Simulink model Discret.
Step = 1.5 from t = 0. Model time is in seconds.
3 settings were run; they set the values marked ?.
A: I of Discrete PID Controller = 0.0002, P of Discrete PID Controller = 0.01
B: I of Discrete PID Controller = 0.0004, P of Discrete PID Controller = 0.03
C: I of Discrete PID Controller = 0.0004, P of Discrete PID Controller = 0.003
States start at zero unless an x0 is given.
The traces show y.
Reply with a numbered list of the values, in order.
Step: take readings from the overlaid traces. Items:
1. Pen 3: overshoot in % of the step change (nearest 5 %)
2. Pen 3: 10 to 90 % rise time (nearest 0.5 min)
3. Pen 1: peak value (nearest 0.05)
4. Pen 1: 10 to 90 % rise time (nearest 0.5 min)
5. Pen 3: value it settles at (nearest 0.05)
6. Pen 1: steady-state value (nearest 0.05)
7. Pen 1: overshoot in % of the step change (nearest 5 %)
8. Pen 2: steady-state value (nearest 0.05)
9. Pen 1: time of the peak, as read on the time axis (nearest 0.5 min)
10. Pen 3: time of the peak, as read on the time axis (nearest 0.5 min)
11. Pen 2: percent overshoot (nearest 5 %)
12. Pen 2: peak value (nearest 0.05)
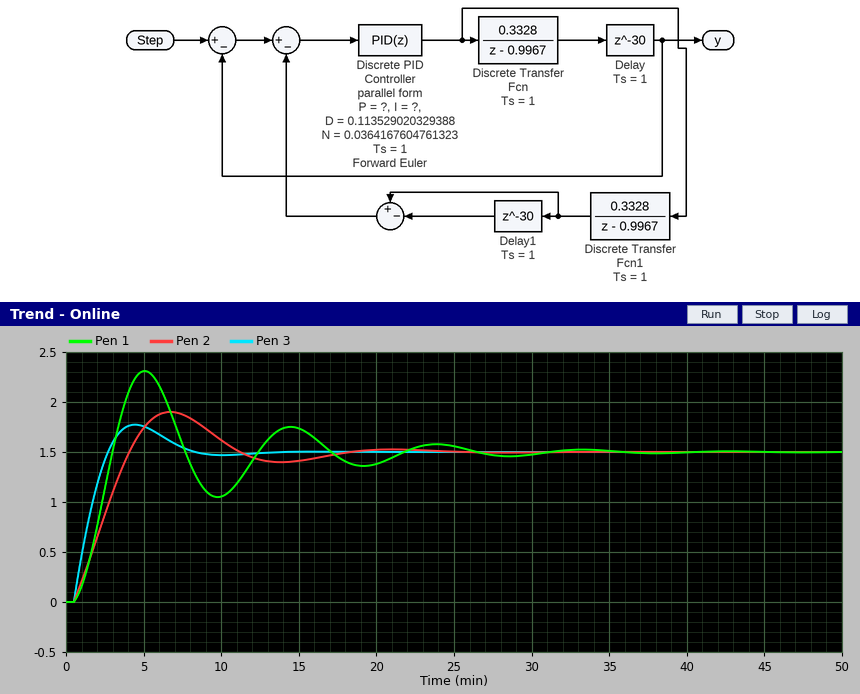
1. 20 %
2. 1.5 min
3. 2.30
4. 2.0 min
5. 1.50
6. 1.50
7. 55 %
8. 1.50
9. 5.0 min
10. 4.5 min
11. 25 %
12. 1.90
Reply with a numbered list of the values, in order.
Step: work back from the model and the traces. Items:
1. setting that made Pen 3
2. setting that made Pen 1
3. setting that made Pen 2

1. B
2. C
3. A
